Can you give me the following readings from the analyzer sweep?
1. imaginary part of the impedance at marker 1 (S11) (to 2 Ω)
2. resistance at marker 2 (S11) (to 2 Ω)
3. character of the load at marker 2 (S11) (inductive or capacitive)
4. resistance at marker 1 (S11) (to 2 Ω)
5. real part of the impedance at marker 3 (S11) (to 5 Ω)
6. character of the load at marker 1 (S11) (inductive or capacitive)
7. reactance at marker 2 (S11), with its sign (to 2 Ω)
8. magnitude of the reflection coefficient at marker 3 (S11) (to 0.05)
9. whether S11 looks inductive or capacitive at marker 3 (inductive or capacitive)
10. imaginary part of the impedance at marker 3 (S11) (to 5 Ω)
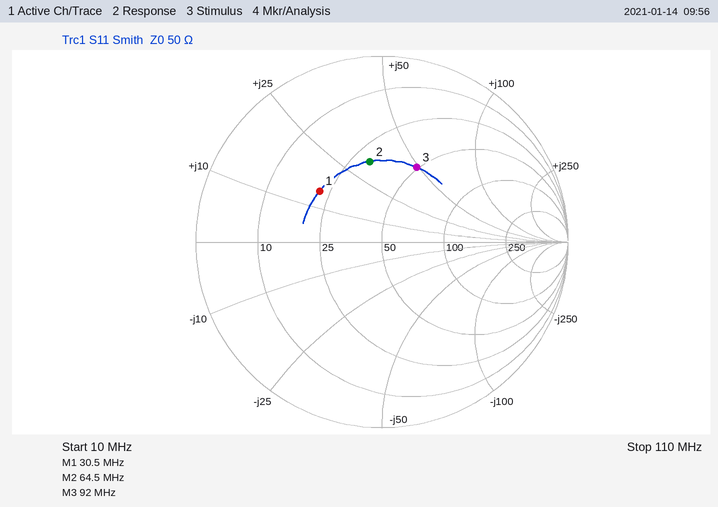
+14 Ω
30 Ω
inductive
22 Ω
50 Ω
inductive
+32 Ω
0.45
inductive
+50 Ω
